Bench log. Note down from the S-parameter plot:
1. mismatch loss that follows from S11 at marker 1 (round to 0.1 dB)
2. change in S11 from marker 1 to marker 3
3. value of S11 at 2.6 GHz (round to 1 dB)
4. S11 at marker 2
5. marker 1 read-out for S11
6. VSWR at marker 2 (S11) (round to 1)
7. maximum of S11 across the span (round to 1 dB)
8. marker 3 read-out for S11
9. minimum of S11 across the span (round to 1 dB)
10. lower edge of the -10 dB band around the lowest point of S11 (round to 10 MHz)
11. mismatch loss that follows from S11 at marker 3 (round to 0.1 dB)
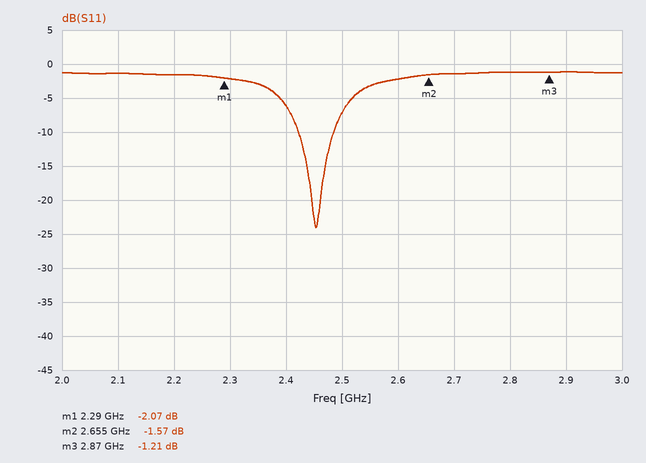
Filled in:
4.2 dB
0.86 dB
-2 dB
-1.57 dB
-2.07 dB
11
-1 dB
-1.21 dB
-24 dB
2.42 GHz
6.1 dB
